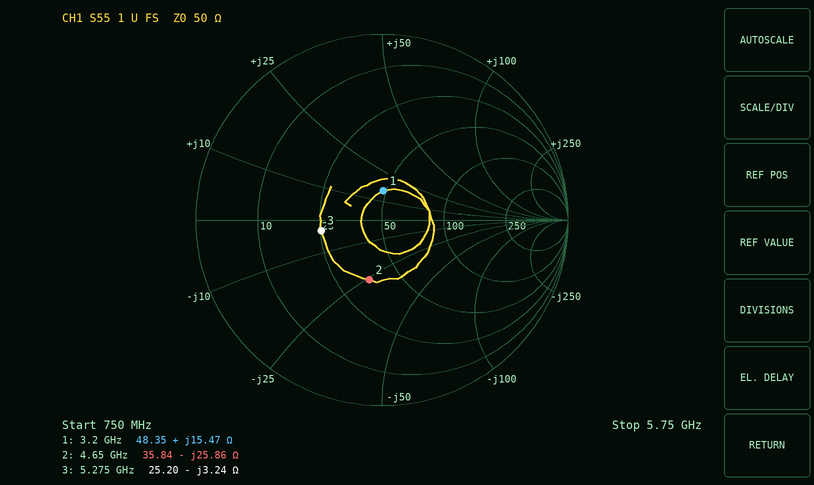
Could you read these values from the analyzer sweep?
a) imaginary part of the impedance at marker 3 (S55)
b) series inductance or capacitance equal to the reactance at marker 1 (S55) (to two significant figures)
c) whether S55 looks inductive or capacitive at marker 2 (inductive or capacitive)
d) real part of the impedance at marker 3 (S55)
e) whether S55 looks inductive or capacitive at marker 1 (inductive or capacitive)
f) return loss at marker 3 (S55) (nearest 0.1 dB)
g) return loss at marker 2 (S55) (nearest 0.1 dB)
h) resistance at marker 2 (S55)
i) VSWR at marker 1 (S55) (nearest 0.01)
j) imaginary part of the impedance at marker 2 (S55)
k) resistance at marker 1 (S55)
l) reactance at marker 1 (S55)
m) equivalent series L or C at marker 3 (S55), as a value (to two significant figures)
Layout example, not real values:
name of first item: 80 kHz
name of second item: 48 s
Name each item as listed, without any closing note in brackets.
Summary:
imaginary part of the impedance at marker 3: -3.24 Ω
series inductance or capacitance equal to the reactance at marker 1 (S55): 770 pH
whether S55 looks inductive or capacitive at marker 2: capacitive
real part of the impedance at marker 3: 25.20 Ω
whether S55 looks inductive or capacitive at marker 1: inductive
return loss at marker 3 (S55): 9.6 dB
return loss at marker 2 (S55): 9.7 dB
resistance at marker 2: 35.84 Ω
VSWR at marker 1 (S55): 1.37
imaginary part of the impedance at marker 2: -25.86 Ω
resistance at marker 1: 48.35 Ω
reactance at marker 1: +15.47 Ω
equivalent series L or C at marker 3 (S55), as a value: 9.3 pF
